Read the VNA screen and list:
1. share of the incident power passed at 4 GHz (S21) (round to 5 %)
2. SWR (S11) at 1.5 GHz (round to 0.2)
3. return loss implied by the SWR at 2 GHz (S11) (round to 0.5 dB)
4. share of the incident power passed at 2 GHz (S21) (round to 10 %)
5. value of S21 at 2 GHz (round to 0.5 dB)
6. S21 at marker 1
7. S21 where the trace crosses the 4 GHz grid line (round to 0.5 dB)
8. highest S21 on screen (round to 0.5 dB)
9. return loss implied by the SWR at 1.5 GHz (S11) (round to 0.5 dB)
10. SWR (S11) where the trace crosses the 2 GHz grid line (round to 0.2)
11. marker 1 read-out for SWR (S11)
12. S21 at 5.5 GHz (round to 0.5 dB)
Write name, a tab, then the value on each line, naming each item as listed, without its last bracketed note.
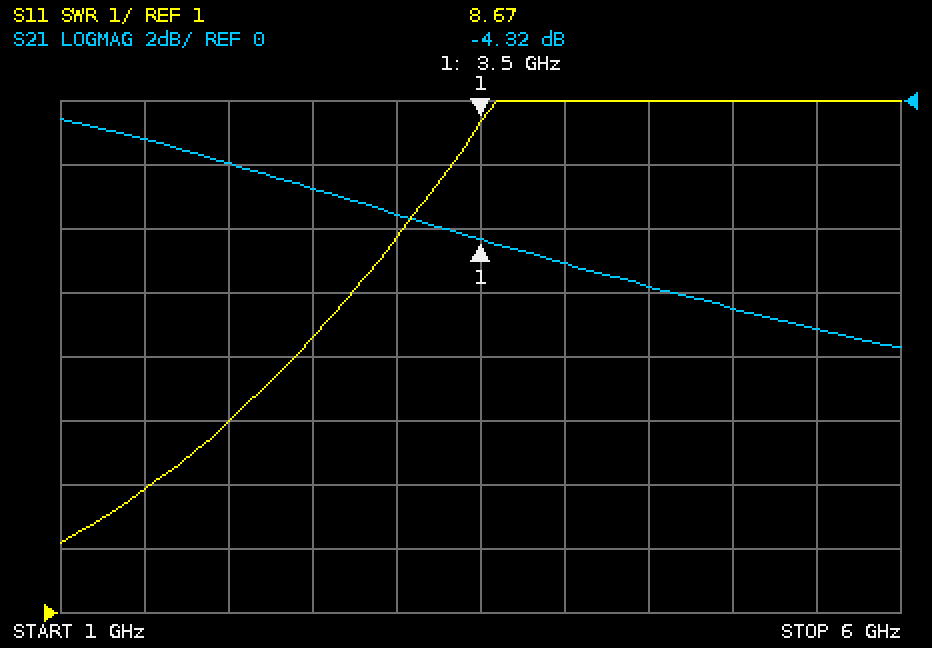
share of the incident power passed at 4 GHz (S21)	30 %
SWR (S11) at 1.5 GHz	3.0
return loss implied by the SWR at 2 GHz (S11)	4.5 dB
share of the incident power passed at 2 GHz (S21)	60 %
value of S21 at 2 GHz	-2.0 dB
S21 at marker 1	-4.32 dB
S21 where the trace crosses the 4 GHz grid line	-5.0 dB
highest S21 on screen	-0.5 dB
return loss implied by the SWR at 1.5 GHz (S11)	6.0 dB
SWR (S11) where the trace crosses the 2 GHz grid line	4.0
marker 1 read-out for SWR	8.67
S21 at 5.5 GHz	-7.0 dB
